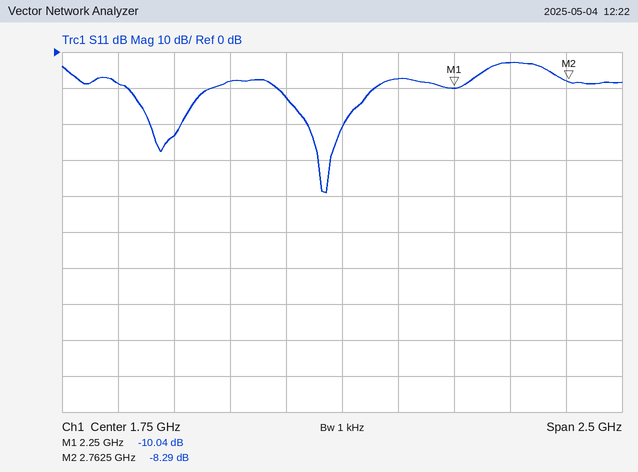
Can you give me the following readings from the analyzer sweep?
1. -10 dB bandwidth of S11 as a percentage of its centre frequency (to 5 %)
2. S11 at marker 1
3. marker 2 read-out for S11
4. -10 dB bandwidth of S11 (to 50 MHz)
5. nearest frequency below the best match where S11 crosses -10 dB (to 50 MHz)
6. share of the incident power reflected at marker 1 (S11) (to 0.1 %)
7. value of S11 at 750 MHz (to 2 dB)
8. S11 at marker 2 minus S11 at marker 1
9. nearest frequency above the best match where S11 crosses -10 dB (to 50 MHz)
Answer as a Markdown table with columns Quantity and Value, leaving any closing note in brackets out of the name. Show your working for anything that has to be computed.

| Quantity | Value |
|---|---|
| -10 dB bandwidth of S11 as a percentage of its centre frequency | 450 MHz / 1.675 GHz ≈ 26.9 %, so 25 % to the nearest 5 % |
| S11 at marker 1 | -10.04 dB |
| marker 2 read-out for S11 | -8.29 dB |
| -10 dB bandwidth of S11 | 1.90 GHz − 1.45 GHz = 450 MHz |
| nearest frequency below the best match where S11 crosses -10 dB | 1.45 GHz |
| share of the incident power reflected at marker 1 (S11) | 10^(-10.04/10) ≈ 9.9 % |
| value of S11 at 750 MHz | -8 dB |
| S11 at marker 2 minus S11 at marker 1 | -8.29 − (-10.04) = 1.75 dB |
| nearest frequency above the best match where S11 crosses -10 dB | 1.90 GHz |
